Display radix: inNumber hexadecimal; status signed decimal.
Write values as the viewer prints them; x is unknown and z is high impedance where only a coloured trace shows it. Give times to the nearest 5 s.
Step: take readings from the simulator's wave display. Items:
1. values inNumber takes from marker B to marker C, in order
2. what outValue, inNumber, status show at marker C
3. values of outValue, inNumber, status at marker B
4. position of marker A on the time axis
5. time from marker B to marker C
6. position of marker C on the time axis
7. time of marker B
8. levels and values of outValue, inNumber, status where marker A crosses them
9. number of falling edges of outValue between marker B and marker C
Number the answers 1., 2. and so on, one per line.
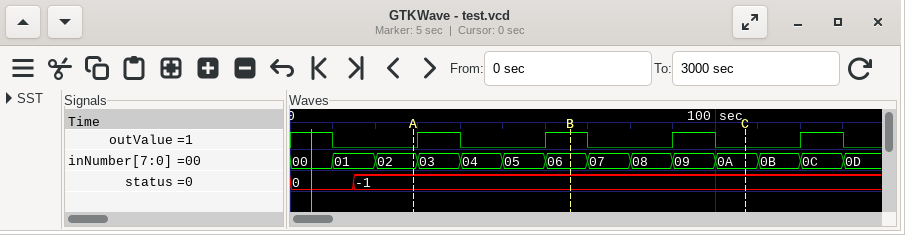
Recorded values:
1. 06, 07, 08, 09, 0A
2. outValue=0, inNumber=0A, status=-1
3. outValue=1, inNumber=06, status=-1
4. 30 s
5. 40 s
6. 105 s
7. 65 s
8. outValue=0, inNumber=02, status=-1
9. 2
